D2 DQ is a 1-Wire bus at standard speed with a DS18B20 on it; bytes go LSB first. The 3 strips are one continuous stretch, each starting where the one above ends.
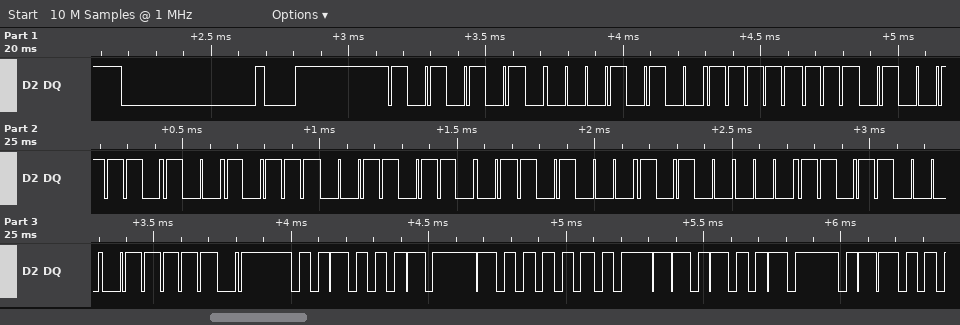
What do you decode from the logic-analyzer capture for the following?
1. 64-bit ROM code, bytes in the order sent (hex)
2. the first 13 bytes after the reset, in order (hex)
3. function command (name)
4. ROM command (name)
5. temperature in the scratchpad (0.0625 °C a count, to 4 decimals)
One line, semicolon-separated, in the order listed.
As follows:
28 FF 72 E9 6C 16 05 1B; 55 28 FF 72 E9 6C 16 05 1B BE 44 01 4B; Read Scratchpad; Match ROM; 20.2500 °C
